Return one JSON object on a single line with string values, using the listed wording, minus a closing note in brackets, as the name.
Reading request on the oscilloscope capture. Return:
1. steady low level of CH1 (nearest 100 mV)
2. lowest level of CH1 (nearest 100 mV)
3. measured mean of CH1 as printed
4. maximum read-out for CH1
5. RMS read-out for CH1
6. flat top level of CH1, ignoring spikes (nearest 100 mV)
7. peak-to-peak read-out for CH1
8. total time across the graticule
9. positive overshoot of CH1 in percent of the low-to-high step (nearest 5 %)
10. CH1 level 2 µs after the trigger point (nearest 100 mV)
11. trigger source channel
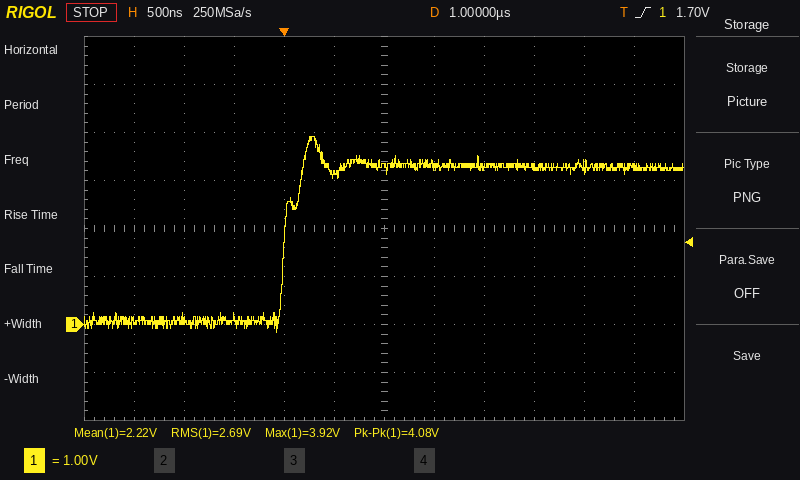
{"steady low level of CH1": "100 mV", "lowest level of CH1": "-200 mV", "measured mean of CH1 as printed": "2.22 V", "maximum read-out for CH1": "3.92 V", "RMS read-out for CH1": "2.69 V", "flat top level of CH1, ignoring spikes": "3.3 V", "peak-to-peak read-out for CH1": "4.08 V", "total time across the graticule": "6 µs", "positive overshoot of CH1 in percent of the low-to-high step": "20 %", "CH1 level 2 µs after the trigger point": "3.3 V", "trigger source channel": "CH1"}
